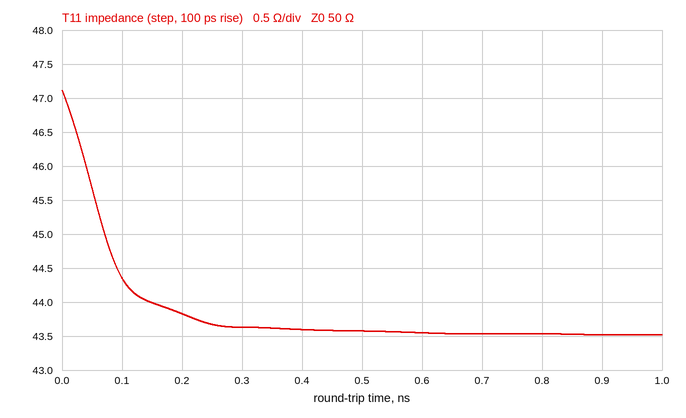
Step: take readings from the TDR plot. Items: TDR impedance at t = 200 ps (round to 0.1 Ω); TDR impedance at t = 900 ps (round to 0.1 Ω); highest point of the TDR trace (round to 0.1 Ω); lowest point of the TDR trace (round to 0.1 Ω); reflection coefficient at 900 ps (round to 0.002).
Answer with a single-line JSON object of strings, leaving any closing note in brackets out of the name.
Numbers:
{"TDR impedance at t = 200 ps": "43.8 Ω", "TDR impedance at t = 900 ps": "43.5 Ω", "highest point of the TDR trace": "47.1 Ω", "lowest point of the TDR trace": "43.5 Ω", "reflection coefficient at 900 ps": "-0.070"}
